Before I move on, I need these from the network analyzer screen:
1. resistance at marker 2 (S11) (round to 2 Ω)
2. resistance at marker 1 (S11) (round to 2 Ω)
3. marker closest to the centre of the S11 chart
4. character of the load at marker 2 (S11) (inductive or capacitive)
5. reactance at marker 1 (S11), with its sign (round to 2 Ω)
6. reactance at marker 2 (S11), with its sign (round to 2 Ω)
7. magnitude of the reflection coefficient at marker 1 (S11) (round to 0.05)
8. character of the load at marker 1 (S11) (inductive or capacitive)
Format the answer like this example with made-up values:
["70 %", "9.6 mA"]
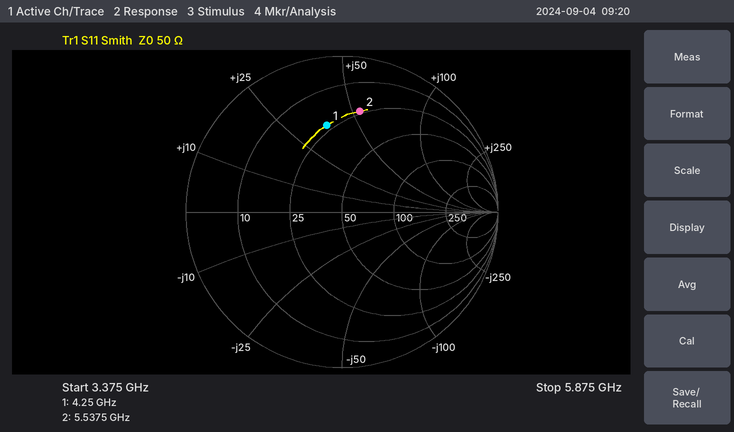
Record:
["24 Ω", "22 Ω", "marker 1", "inductive", "+36 Ω", "+54 Ω", "0.55", "inductive"]
